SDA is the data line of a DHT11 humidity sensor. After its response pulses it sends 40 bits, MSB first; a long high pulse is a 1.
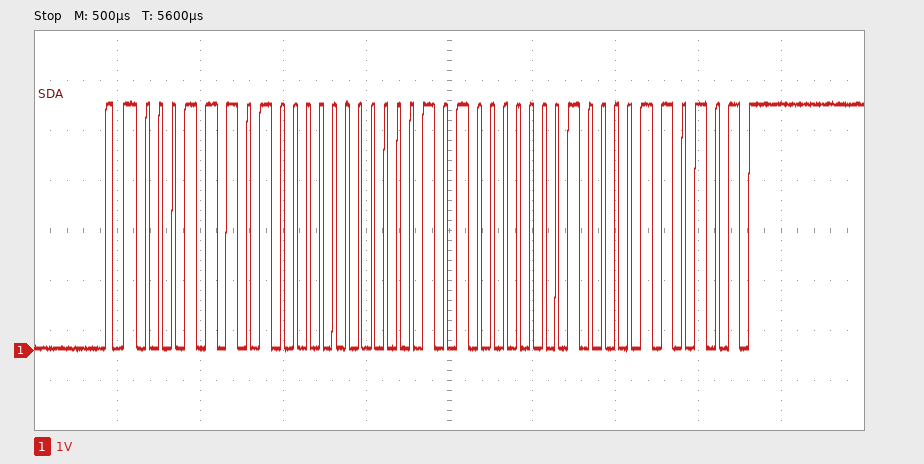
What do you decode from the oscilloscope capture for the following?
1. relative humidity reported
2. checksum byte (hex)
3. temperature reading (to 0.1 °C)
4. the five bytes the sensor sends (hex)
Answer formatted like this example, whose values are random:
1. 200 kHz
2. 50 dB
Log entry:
1. 29 %
2. 0x35
3. 20.4 °C
4. 1D 00 14 04 35
